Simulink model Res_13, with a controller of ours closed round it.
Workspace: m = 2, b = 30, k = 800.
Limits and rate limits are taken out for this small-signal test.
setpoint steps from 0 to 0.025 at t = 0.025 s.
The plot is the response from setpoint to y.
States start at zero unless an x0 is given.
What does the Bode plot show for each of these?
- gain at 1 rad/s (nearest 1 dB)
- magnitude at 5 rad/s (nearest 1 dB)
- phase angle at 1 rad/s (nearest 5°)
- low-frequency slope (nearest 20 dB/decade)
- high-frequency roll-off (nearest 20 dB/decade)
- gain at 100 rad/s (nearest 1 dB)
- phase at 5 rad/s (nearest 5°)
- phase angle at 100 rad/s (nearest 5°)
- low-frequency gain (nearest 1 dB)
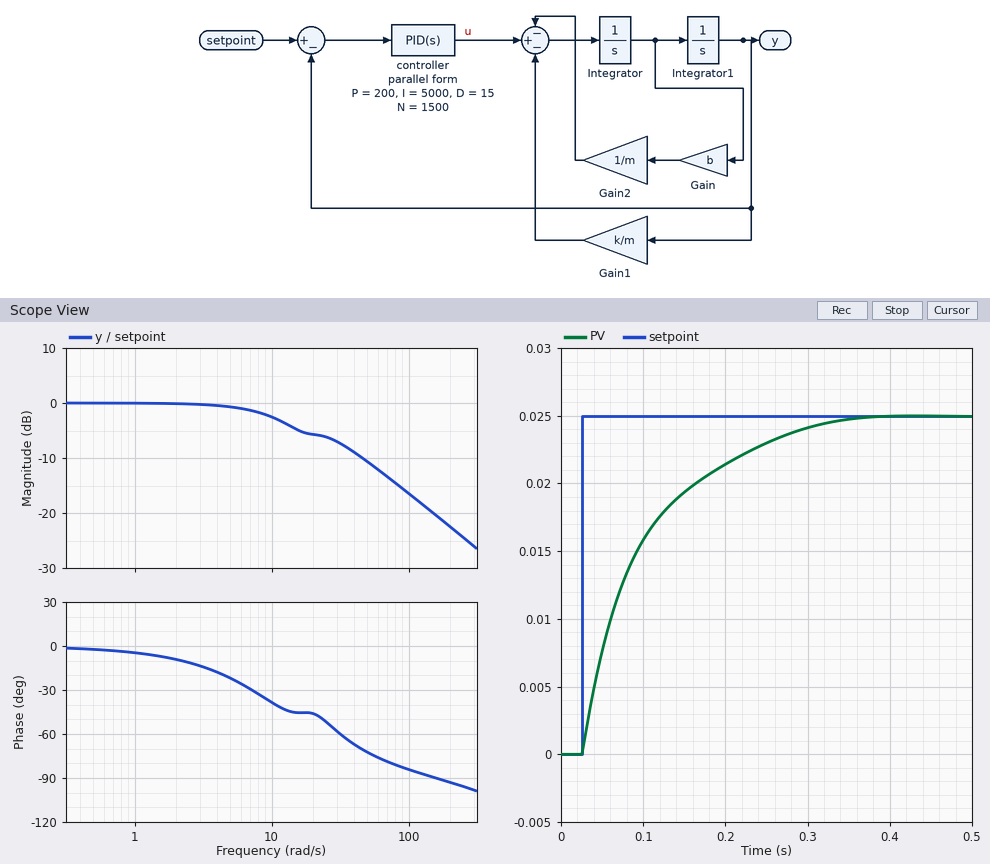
0 dB
-1 dB
-5°
0 dB/decade
-20 dB/decade
-16 dB
-20°
-85°
0 dB
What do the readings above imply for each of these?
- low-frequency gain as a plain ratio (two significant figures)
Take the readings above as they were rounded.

1.0
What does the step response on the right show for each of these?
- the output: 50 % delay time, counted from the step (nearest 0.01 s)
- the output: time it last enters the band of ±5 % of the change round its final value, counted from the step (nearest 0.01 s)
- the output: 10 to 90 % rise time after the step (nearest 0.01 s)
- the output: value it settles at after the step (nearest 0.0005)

0.05 s
0.26 s
0.20 s
0.0250
